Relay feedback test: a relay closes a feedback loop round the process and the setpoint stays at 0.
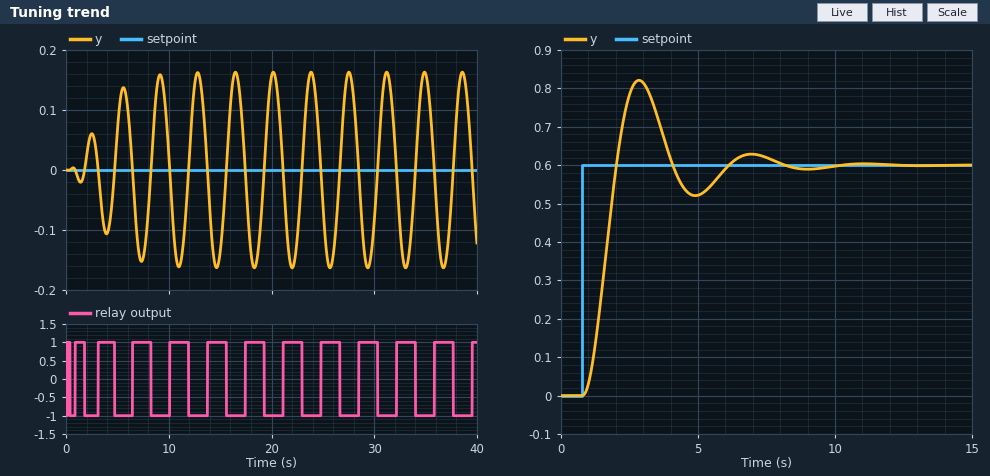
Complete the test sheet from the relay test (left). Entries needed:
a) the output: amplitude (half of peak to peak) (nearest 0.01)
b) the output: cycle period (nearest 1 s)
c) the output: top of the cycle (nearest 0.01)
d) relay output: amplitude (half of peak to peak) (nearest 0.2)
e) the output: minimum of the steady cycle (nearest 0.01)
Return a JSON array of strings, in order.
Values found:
["0.16", "4 s", "0.16", "1.0", "-0.16"]
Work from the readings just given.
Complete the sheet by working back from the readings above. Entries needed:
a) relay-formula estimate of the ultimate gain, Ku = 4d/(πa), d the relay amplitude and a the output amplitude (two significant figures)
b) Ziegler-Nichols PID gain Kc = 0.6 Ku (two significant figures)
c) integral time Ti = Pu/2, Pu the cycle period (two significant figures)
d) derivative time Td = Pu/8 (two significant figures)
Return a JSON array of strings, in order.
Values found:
["8.0", "4.8", "2.0 s", "0.50 s"]
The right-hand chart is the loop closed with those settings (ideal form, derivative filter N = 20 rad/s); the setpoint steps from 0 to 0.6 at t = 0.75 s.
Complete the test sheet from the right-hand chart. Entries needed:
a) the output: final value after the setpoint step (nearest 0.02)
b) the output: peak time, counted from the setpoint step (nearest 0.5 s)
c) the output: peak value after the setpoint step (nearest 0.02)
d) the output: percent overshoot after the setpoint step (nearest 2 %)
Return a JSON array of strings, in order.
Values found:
["0.60", "2.0 s", "0.82", "36 %"]
